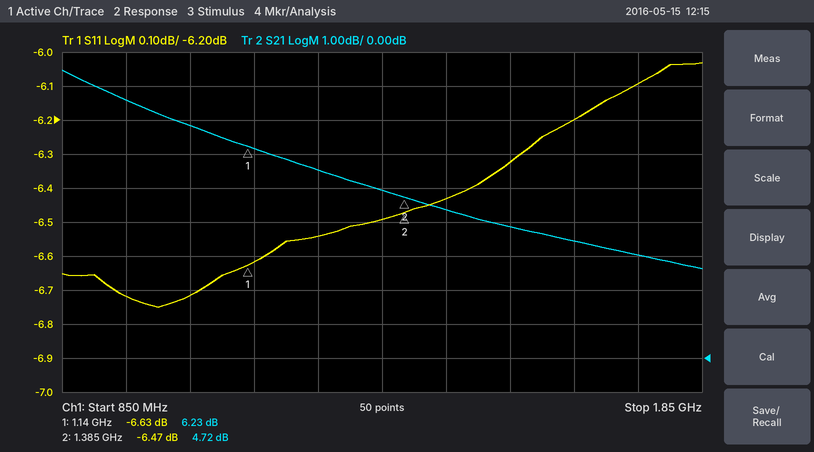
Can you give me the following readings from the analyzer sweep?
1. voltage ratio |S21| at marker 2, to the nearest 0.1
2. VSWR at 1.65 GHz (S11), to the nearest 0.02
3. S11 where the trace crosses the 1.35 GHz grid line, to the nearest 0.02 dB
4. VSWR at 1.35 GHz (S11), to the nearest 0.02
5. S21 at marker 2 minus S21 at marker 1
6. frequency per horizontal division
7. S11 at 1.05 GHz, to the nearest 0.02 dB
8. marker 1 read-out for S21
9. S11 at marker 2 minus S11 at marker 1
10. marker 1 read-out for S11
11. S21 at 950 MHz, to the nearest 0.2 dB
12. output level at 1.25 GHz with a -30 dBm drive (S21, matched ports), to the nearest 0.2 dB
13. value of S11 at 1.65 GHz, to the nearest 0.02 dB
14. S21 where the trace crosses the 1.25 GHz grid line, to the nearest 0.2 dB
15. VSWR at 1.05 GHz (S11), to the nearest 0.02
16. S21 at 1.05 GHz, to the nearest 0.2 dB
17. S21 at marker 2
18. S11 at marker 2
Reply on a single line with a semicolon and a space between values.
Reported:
1.7; 2.92; -6.50 dB; 2.80; -1.51 dB; 100 MHz; -6.72 dB; 6.23 dB; 0.16 dB; -6.63 dB; 7.6 dB; -24.4 dBm; -6.20 dB; 5.6 dB; 2.72; 6.8 dB; 4.72 dB; -6.47 dB
